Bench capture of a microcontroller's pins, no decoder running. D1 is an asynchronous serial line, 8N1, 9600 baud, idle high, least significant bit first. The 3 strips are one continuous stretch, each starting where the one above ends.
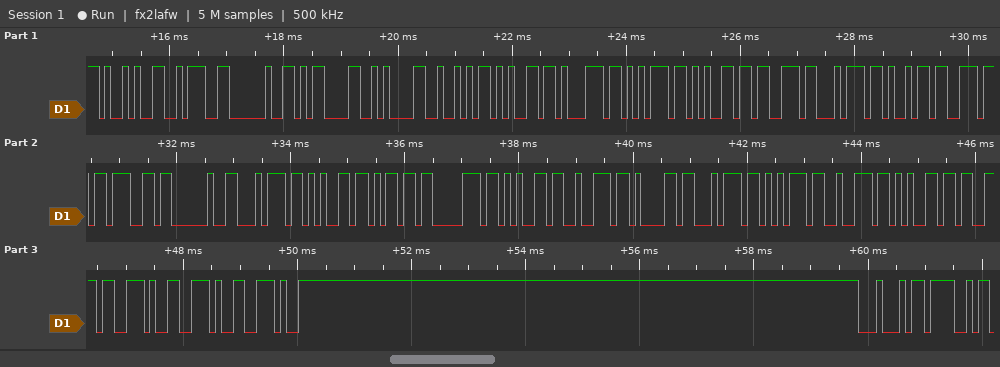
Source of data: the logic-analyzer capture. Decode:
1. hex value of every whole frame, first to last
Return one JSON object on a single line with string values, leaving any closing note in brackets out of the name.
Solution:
{"hex value of every whole frame, first to last": "29 3A 20 0D 0A 52 65 71 75 65 73 74 69 6E 67 20 74 65 6D 70 65 72 61 74 75 72 65 73 2E 2E 2E 44 4F"}
